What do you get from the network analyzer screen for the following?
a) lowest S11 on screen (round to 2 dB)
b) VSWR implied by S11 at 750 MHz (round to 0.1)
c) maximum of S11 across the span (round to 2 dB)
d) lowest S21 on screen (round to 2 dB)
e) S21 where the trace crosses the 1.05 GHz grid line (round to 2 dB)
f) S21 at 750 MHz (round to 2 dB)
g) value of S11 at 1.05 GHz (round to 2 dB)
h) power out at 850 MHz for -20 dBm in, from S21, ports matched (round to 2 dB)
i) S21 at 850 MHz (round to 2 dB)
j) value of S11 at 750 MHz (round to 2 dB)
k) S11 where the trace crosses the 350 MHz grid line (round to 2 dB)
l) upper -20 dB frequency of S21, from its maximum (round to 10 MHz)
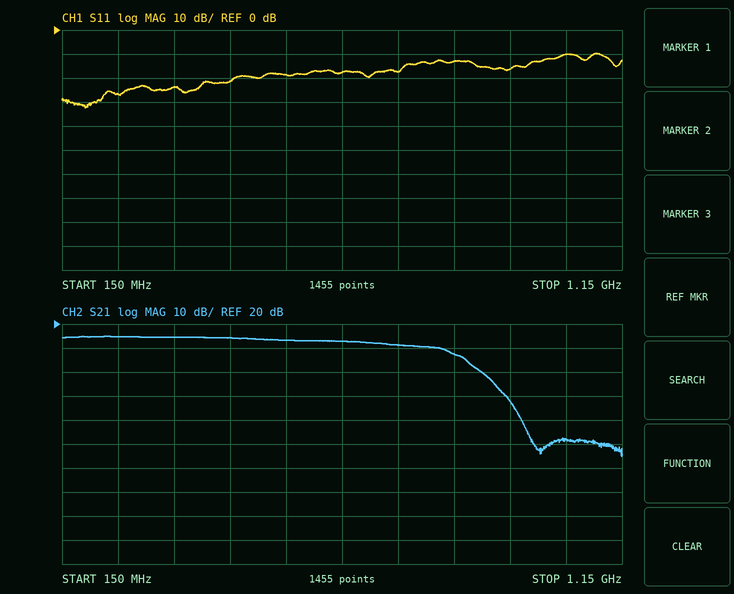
-32 dB
1.3
-10 dB
-36 dB
-28 dB
12 dB
-10 dB
-12 dBm
8 dB
-18 dB
-24 dB
920 MHz
